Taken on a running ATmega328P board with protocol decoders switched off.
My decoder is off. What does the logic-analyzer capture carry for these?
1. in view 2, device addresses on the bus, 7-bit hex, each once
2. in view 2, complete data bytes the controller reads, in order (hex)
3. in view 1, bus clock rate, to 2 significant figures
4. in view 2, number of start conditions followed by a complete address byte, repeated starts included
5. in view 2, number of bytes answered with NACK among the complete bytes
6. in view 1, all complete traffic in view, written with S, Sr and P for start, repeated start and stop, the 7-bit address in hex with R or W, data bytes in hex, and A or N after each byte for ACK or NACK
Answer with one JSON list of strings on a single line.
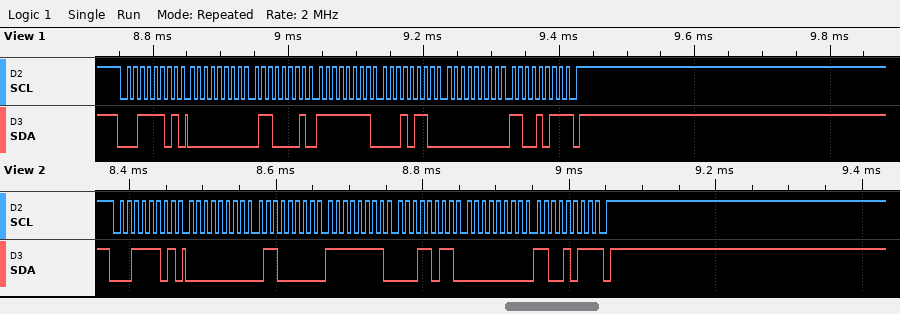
["0x1E", "00 60 FF 1B 00 CB", "100 kHz", "1", "1", "S 1ER A 00 A 61 A FF A 16 A 00 A CB N P"]
